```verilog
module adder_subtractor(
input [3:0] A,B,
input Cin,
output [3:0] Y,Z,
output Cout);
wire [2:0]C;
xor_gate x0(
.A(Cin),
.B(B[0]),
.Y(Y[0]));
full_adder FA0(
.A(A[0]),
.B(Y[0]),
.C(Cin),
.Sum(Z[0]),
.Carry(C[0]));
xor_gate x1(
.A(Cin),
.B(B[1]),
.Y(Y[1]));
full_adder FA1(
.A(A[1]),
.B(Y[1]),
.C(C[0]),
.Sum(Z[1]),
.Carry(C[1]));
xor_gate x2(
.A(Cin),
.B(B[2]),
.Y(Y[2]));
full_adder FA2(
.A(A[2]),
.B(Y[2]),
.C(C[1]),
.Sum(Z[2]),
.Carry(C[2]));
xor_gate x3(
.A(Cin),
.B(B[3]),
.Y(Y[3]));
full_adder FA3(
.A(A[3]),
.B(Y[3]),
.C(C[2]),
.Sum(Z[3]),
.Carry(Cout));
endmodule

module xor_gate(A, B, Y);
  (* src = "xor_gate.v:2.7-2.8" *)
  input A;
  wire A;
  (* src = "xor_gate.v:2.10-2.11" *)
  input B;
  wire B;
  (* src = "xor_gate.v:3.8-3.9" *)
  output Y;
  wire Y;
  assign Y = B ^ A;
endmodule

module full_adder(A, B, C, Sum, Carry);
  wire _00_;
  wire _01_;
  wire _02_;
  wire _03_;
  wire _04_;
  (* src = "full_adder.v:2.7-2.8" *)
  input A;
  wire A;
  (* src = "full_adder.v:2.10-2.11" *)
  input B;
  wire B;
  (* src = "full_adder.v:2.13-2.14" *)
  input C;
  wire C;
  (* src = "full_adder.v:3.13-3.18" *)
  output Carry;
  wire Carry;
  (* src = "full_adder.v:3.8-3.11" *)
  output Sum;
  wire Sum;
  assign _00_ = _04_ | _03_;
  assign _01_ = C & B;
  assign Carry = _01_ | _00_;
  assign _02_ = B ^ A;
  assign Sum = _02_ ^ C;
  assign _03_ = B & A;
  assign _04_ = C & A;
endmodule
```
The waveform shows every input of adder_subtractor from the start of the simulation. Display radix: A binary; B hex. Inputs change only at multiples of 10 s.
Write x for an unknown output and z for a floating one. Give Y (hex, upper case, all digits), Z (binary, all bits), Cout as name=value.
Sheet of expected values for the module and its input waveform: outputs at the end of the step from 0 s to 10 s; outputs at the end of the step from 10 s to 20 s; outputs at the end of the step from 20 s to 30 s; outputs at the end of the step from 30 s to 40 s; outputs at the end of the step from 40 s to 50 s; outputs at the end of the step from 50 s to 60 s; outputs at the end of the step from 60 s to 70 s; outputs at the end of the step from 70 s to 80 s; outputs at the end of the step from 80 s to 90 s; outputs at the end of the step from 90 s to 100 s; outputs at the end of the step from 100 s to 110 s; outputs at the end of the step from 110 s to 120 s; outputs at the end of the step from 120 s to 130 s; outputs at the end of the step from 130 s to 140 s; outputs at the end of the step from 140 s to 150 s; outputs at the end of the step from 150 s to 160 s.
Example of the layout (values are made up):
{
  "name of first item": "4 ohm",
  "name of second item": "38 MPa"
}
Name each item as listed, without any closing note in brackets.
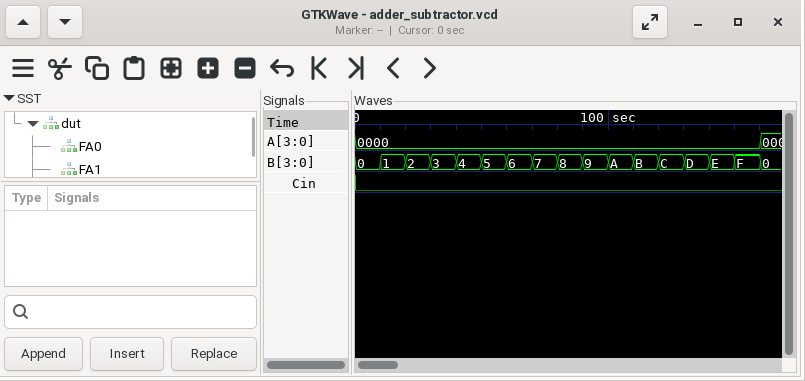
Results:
{
  "outputs at the end of the step from 0 s to 10 s": "Y=0, Z=0000, Cout=0",
  "outputs at the end of the step from 10 s to 20 s": "Y=1, Z=0001, Cout=0",
  "outputs at the end of the step from 20 s to 30 s": "Y=2, Z=0010, Cout=0",
  "outputs at the end of the step from 30 s to 40 s": "Y=3, Z=0011, Cout=0",
  "outputs at the end of the step from 40 s to 50 s": "Y=4, Z=0100, Cout=0",
  "outputs at the end of the step from 50 s to 60 s": "Y=5, Z=0101, Cout=0",
  "outputs at the end of the step from 60 s to 70 s": "Y=6, Z=0110, Cout=0",
  "outputs at the end of the step from 70 s to 80 s": "Y=7, Z=0111, Cout=0",
  "outputs at the end of the step from 80 s to 90 s": "Y=8, Z=1000, Cout=0",
  "outputs at the end of the step from 90 s to 100 s": "Y=9, Z=1001, Cout=0",
  "outputs at the end of the step from 100 s to 110 s": "Y=A, Z=1010, Cout=0",
  "outputs at the end of the step from 110 s to 120 s": "Y=B, Z=1011, Cout=0",
  "outputs at the end of the step from 120 s to 130 s": "Y=C, Z=1100, Cout=0",
  "outputs at the end of the step from 130 s to 140 s": "Y=D, Z=1101, Cout=0",
  "outputs at the end of the step from 140 s to 150 s": "Y=E, Z=1110, Cout=0",
  "outputs at the end of the step from 150 s to 160 s": "Y=F, Z=1111, Cout=0"
}
